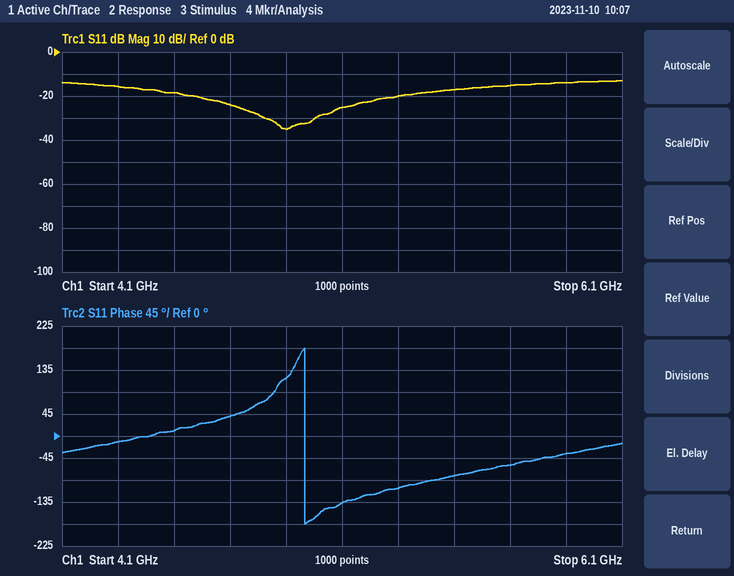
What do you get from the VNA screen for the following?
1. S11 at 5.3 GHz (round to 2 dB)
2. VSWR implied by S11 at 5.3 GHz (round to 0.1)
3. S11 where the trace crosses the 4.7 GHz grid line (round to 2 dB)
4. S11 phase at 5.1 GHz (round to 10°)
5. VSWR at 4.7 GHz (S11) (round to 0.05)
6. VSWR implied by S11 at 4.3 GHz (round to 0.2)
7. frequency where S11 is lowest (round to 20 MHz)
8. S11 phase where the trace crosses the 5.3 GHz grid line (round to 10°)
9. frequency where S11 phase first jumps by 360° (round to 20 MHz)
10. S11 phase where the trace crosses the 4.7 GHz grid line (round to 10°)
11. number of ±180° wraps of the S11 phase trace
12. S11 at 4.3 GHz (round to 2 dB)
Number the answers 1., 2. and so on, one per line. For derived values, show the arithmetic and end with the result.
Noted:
1. -20 dB
2. |Γ| = 10^(-20/20) = 0.1000; VSWR = (1 + 0.1000)/(1 − 0.1000) ≈ 1.2
3. -24 dB
4. -140°
5. |Γ| = 10^(-24/20) = 0.0631; VSWR = (1 + 0.0631)/(1 − 0.0631) ≈ 1.13, so 1.15 to the nearest 0.05
6. |Γ| = 10^(-16/20) = 0.1585; VSWR = (1 + 0.1585)/(1 − 0.1585) ≈ 1.4
7. 4.90 GHz
8. -110°
9. 4.96 GHz
10. 40°
11. 1
12. -16 dB
